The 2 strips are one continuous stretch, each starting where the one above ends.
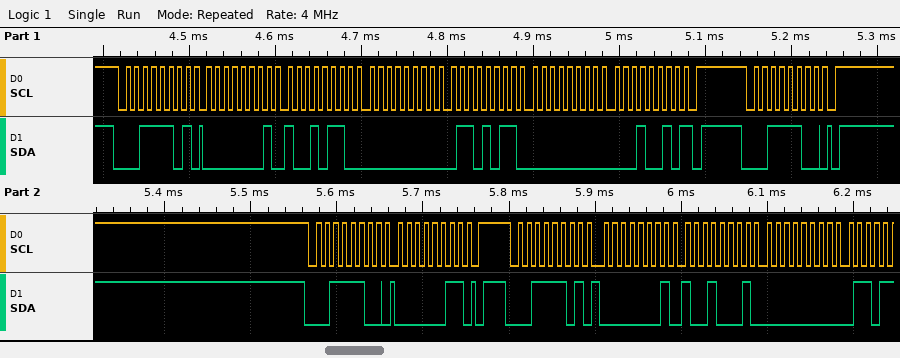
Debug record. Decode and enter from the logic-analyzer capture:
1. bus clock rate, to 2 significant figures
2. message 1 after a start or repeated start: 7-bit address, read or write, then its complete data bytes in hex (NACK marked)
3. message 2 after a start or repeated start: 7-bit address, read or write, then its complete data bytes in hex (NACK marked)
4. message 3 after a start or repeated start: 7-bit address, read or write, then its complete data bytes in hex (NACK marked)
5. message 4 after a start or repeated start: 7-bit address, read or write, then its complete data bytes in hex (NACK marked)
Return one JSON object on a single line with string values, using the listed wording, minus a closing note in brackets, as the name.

{"bus clock rate, to 2 significant figures": "100 kHz", "message 1 after a start or repeated start: 7-bit address, read or write, then its complete data bytes in hex": "0x1E read: 01 96 00 6B 00 12 NACK", "message 2 after a start or repeated start: 7-bit address, read or write, then its complete data bytes in hex": "0x1E write", "message 3 after a start or repeated start: 7-bit address, read or write, then its complete data bytes in hex": "0x1E write: 03", "message 4 after a start or repeated start: 7-bit address, read or write, then its complete data bytes in hex": "0x1E read: 01 91 00"}
